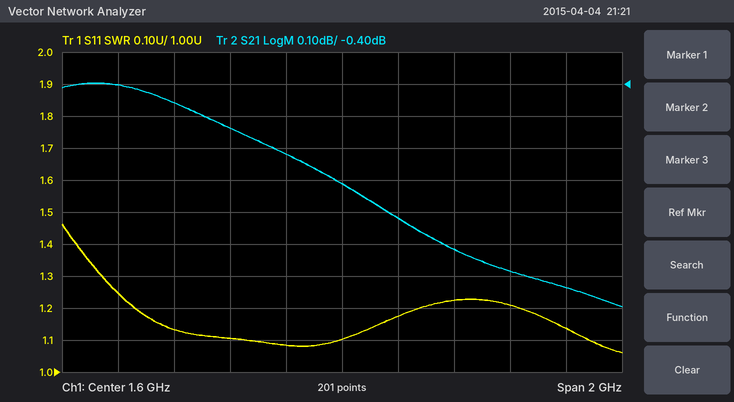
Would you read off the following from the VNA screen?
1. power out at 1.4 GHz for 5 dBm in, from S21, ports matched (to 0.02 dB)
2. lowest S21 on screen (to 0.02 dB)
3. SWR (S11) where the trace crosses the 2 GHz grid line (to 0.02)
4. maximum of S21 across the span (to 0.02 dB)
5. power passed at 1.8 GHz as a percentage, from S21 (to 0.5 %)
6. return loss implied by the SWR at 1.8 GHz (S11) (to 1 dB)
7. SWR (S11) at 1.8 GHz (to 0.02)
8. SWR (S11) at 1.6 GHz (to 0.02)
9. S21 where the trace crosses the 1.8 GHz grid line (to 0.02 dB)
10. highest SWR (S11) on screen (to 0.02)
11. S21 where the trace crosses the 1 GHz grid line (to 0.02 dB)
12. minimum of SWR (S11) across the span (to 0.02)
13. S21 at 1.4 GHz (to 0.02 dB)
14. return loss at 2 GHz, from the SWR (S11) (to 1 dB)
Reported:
4.38 dBm
-1.10 dB
1.22
-0.40 dB
83.0 %
22 dB
1.18
1.10
-0.82 dB
1.46
-0.46 dB
1.06
-0.62 dB
20 dB
